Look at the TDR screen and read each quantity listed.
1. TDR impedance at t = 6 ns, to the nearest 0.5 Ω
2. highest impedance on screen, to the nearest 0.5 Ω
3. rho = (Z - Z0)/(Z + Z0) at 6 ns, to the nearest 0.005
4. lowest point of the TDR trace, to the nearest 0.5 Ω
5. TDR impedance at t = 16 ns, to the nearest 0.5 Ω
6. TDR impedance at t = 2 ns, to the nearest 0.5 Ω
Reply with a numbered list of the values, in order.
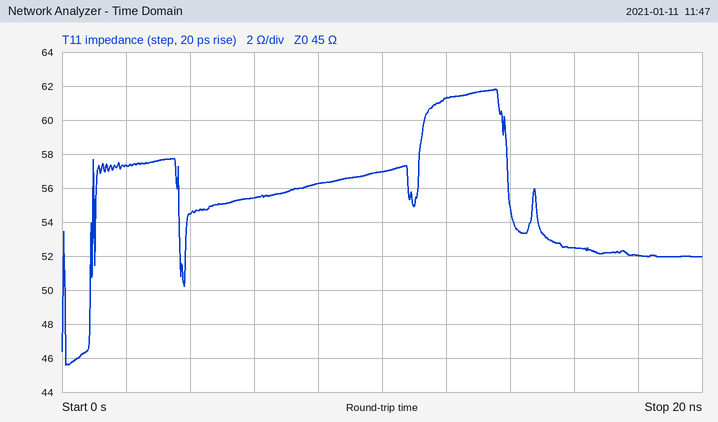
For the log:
1. 55.5 Ω
2. 62.0 Ω
3. +0.105
4. 45.5 Ω
5. 52.5 Ω
6. 57.5 Ω
